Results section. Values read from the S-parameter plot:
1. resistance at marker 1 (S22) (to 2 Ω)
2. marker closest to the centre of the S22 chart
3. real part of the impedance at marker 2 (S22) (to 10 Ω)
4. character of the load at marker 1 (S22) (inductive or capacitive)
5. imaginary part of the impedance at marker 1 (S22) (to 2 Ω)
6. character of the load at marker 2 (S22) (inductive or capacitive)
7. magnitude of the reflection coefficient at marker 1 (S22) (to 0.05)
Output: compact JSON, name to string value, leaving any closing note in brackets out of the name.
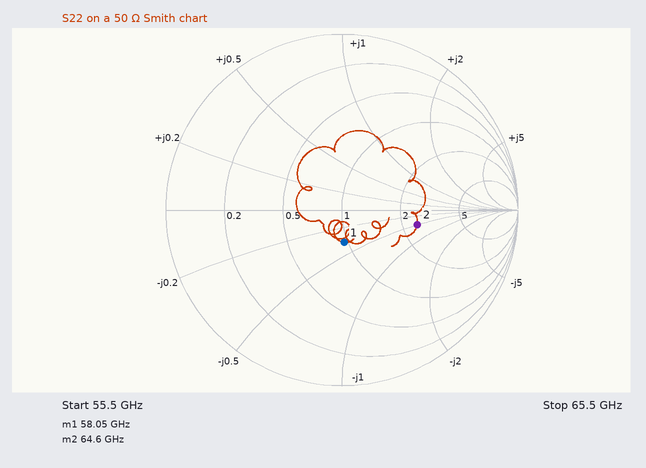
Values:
{"resistance at marker 1 (S22)": "48 Ω", "marker closest to the centre of the S22 chart": "marker 1", "real part of the impedance at marker 2 (S22)": "120 Ω", "character of the load at marker 1 (S22)": "capacitive", "imaginary part of the impedance at marker 1 (S22)": "-18 Ω", "character of the load at marker 2 (S22)": "capacitive", "magnitude of the reflection coefficient at marker 1 (S22)": "0.20"}
